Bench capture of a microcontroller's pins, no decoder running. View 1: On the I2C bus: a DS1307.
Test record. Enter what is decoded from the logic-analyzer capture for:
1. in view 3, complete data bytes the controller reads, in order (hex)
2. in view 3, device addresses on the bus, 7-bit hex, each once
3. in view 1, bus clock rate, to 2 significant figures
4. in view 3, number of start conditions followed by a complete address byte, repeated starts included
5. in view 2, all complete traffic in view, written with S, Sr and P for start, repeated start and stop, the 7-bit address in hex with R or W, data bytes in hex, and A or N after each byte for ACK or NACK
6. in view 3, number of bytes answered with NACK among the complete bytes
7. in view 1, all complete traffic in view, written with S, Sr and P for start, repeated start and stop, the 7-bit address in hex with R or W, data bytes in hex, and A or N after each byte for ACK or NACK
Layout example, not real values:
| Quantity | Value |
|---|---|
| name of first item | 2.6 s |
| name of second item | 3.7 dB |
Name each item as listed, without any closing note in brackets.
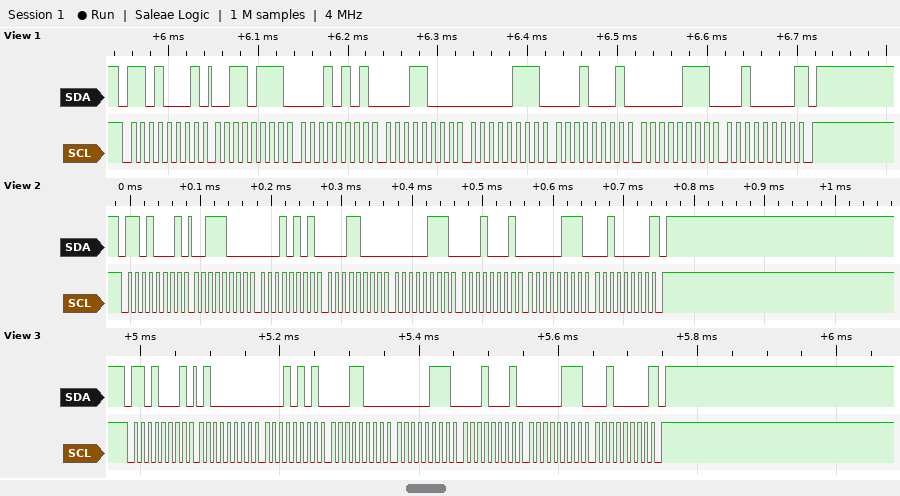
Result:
| Quantity | Value |
|---|---|
| in view 3, complete data bytes the controller reads, in order | 40 15 18 07 11 07 20 |
| in view 3, device addresses on the bus, 7-bit hex, each once | 0x68 |
| in view 1, bus clock rate, to 2 significant figures | 100 kHz |
| in view 3, number of start conditions followed by a complete address byte, repeated starts included | 1 |
| in view 2, all complete traffic in view, written with S, Sr and P for start, repeated start and stop, the 7-bit address in hex with R or W, data bytes in hex, and A or N after each byte for ACK or NACK | S 68R A 38 A 15 A 18 A 07 A 11 A 07 A 20 N P |
| in view 3, number of bytes answered with NACK among the complete bytes | 1 |
| in view 1, all complete traffic in view, written with S, Sr and P for start, repeated start and stop, the 7-bit address in hex with R or W, data bytes in hex, and A or N after each byte for ACK or NACK | S 68R A 37 A 15 A 18 A 07 A 11 A 07 A 20 N P |
